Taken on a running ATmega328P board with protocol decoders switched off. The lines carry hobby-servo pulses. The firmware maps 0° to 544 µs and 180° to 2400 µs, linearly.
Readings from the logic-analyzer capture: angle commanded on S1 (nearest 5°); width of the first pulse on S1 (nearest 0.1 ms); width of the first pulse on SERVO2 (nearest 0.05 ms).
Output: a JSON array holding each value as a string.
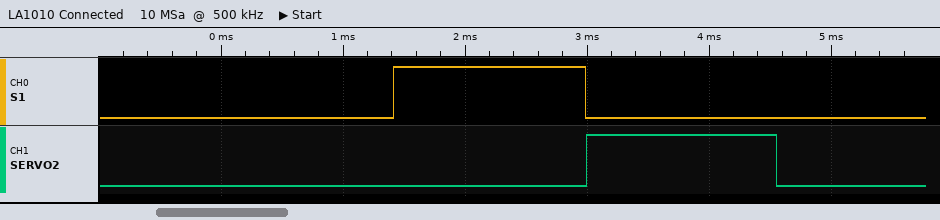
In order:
["100°", "1.6 ms", "1.55 ms"]
